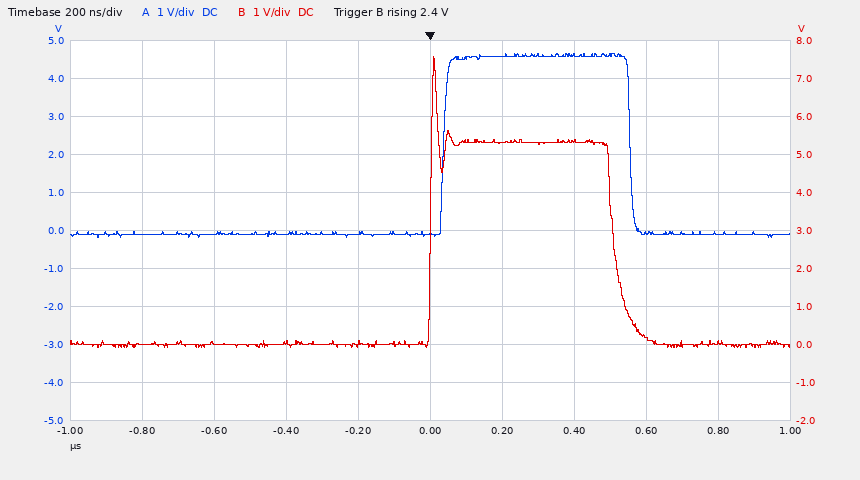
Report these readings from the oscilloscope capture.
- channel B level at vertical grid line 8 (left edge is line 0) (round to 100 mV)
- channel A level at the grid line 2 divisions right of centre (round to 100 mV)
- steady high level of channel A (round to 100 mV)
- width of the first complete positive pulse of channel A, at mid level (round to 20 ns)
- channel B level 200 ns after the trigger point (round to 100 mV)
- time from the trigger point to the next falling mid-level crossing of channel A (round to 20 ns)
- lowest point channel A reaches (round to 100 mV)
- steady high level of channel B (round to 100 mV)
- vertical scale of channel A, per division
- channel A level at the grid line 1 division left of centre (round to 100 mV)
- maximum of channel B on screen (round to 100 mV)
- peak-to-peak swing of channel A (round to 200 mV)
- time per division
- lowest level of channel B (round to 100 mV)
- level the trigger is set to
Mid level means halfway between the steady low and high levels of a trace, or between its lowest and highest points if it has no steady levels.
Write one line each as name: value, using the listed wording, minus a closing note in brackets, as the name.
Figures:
channel B level at vertical grid line 8 (left edge is line 0): 200 mV
channel A level at the grid line 2 divisions right of centre: 4.6 V
steady high level of channel A: 4.6 V
width of the first complete positive pulse of channel A, at mid level: 520 ns
channel B level 200 ns after the trigger point: 5.3 V
time from the trigger point to the next falling mid-level crossing of channel A: 560 ns
lowest point channel A reaches: -200 mV
steady high level of channel B: 5.3 V
vertical scale of channel A, per division: 1 V
channel A level at the grid line 1 division left of centre: -100 mV
maximum of channel B on screen: 7.6 V
peak-to-peak swing of channel A: 4.8 V
time per division: 200 ns
lowest level of channel B: -100 mV
level the trigger is set to: 2.4 V
